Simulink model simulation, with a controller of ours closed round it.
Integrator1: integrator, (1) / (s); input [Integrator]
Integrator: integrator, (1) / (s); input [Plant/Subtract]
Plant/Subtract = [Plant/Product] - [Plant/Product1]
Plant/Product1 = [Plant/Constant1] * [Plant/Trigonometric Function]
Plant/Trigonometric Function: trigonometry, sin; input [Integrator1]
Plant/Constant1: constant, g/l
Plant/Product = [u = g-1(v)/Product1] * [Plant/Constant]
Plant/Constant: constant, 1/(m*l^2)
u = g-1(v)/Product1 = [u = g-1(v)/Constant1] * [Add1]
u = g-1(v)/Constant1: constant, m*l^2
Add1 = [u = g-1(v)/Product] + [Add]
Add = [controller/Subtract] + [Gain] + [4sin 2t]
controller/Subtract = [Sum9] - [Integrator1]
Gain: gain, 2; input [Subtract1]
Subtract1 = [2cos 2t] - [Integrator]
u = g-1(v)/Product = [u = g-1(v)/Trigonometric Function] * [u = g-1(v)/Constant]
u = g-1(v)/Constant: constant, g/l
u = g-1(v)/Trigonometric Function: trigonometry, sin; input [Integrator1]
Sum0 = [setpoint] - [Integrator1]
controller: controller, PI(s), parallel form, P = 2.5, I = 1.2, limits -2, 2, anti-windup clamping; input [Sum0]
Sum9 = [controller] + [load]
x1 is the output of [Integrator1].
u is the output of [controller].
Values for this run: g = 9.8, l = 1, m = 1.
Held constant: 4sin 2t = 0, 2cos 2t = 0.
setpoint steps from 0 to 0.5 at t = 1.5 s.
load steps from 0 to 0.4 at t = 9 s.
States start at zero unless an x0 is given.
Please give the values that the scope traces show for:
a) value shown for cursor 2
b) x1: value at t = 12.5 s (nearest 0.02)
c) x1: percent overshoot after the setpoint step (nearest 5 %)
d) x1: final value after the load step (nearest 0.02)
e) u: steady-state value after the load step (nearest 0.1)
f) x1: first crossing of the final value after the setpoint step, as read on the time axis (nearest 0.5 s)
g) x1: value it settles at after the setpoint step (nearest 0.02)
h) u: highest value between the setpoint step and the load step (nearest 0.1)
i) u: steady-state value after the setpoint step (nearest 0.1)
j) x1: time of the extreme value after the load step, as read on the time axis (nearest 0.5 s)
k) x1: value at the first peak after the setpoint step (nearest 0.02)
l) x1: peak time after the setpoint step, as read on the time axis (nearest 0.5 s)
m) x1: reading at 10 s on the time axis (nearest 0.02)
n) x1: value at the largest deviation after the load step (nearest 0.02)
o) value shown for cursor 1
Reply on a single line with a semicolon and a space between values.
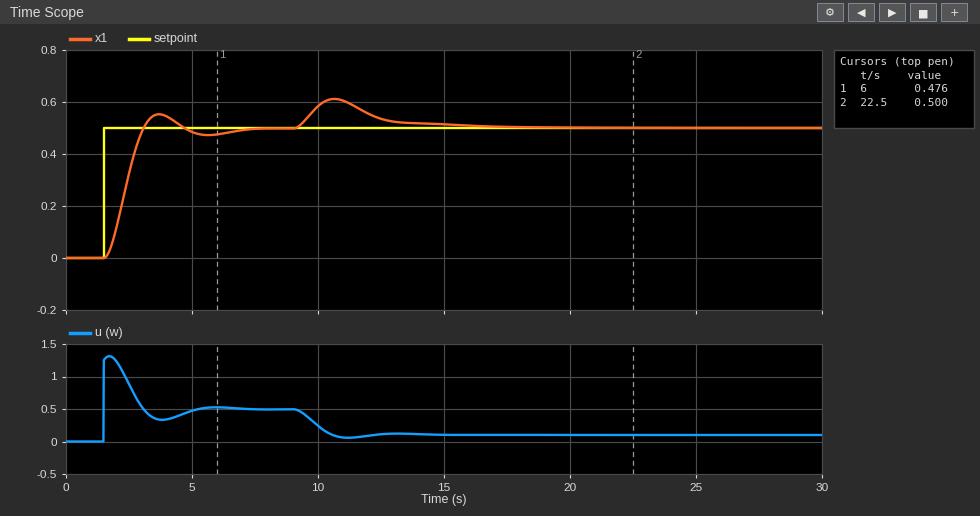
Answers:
0.500; 0.54; 10 %; 0.50; 0.1; 3.0 s; 0.50; 1.3; 0.5; 10.5 s; 0.56; 3.5 s; 0.58; 0.62; 0.476
